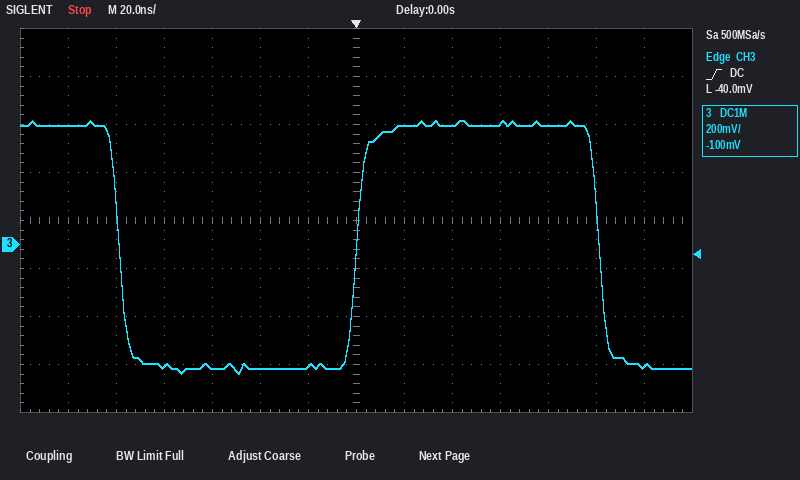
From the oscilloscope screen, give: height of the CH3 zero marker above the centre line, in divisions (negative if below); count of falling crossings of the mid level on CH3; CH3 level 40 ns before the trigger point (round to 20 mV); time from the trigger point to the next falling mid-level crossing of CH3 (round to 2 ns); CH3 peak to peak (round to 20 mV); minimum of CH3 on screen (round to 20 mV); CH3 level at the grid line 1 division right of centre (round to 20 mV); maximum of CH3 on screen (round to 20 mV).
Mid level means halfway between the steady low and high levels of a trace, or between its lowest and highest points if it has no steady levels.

-0.5 div
2
-520 mV
102 ns
1.06 V
-540 mV
500 mV
520 mV
